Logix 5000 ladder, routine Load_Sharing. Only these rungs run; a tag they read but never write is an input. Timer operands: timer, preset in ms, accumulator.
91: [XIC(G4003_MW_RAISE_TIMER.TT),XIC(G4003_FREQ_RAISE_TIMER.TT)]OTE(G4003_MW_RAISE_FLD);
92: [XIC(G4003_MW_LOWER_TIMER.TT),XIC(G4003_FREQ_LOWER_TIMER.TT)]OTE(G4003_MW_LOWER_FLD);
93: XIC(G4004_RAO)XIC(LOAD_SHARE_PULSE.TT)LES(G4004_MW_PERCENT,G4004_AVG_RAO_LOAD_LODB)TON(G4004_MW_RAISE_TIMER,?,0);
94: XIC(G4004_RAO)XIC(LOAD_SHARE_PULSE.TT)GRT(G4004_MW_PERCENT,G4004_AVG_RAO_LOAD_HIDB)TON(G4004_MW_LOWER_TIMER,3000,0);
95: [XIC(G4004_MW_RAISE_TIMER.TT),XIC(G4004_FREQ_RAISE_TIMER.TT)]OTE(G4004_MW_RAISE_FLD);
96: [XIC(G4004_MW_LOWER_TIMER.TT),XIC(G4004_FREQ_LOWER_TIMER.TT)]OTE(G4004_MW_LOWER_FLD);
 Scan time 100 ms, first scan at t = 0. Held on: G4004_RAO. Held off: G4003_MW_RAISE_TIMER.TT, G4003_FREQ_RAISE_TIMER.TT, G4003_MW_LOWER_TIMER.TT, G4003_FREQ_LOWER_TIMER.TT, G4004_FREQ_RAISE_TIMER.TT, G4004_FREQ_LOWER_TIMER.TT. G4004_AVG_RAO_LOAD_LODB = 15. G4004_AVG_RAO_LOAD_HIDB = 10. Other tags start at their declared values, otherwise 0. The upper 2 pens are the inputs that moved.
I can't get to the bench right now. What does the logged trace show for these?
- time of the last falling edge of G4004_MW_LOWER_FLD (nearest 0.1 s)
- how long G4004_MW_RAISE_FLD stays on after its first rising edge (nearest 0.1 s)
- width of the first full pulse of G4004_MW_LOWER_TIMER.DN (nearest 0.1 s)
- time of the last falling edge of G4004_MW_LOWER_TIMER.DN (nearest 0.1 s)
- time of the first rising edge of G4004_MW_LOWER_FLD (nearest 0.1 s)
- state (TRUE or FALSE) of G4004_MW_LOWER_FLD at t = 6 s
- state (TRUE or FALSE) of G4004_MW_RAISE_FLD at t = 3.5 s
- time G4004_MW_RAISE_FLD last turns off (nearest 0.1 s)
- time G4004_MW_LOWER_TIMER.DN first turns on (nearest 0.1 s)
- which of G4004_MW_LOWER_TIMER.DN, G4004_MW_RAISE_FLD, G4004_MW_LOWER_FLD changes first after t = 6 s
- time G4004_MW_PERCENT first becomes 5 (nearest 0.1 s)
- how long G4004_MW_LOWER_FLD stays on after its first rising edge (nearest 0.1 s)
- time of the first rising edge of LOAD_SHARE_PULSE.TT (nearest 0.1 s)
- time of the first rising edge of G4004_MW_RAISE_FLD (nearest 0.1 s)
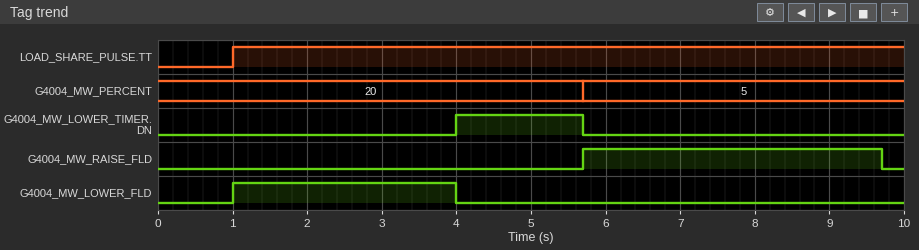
4.0 s
4.0 s
1.7 s
5.7 s
1.0 s
FALSE
FALSE
9.7 s
4.0 s
G4004_MW_RAISE_FLD
5.7 s
3.0 s
1.0 s
5.7 s
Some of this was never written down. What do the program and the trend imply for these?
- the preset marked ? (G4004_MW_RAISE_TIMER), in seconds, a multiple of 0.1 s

4.0 s
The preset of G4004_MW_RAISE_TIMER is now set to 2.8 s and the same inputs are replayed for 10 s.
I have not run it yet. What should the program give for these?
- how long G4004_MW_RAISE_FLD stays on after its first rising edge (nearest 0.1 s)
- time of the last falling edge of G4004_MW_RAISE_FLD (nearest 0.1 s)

2.8 s
8.5 s
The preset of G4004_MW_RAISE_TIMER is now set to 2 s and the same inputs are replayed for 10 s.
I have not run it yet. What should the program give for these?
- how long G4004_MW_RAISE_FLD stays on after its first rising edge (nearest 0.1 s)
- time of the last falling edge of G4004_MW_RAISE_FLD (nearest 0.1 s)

2.0 s
7.7 s
